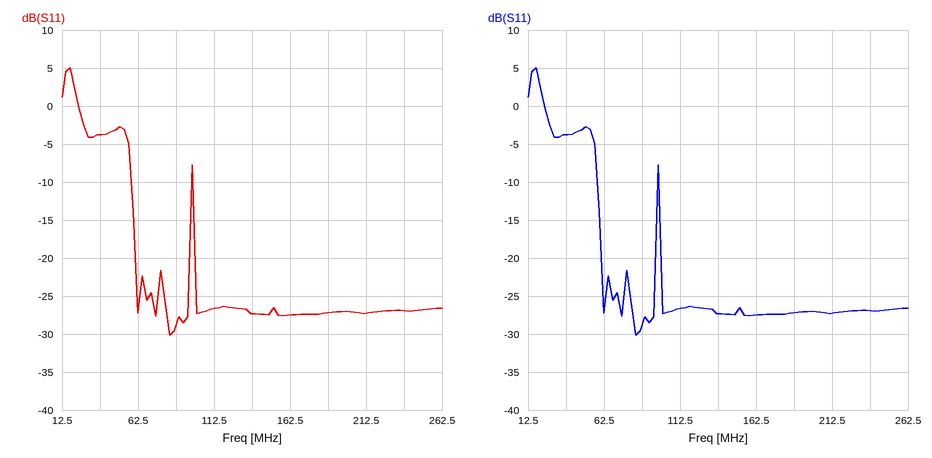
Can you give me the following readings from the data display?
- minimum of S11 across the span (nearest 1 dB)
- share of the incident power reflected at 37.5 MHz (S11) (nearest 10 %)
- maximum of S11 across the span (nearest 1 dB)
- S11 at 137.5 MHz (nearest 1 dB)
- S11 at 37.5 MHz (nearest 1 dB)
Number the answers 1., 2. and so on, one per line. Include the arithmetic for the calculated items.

1. -30 dB
2. 10^(-4/10) ≈ 40 %
3. 5 dB
4. -27 dB
5. -4 dB
